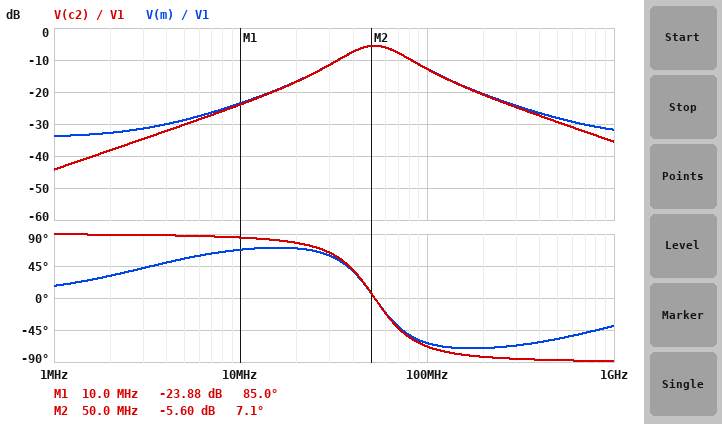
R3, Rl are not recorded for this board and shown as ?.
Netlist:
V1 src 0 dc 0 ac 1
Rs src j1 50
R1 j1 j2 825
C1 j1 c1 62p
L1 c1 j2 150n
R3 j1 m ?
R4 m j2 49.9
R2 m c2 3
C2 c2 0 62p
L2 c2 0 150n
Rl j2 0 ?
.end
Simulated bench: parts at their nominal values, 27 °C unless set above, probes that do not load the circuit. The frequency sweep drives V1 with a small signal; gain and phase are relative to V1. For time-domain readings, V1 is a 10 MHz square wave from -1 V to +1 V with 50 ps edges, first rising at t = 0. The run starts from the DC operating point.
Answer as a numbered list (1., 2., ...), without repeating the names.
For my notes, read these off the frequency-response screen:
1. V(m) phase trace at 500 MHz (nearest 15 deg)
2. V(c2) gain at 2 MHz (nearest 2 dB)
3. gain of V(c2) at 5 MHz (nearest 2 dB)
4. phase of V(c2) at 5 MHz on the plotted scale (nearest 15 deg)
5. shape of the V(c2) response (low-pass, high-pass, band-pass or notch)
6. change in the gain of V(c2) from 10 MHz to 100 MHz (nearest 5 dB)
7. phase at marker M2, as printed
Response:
1. -60 deg
2. -38 dB
3. -30 dB
4. 90 deg
5. band-pass
6. 10 dB
7. 7.1 deg
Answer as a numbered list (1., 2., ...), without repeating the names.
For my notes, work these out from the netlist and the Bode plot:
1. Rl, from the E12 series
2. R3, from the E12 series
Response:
1. 56 Ω
2. 100 Ω
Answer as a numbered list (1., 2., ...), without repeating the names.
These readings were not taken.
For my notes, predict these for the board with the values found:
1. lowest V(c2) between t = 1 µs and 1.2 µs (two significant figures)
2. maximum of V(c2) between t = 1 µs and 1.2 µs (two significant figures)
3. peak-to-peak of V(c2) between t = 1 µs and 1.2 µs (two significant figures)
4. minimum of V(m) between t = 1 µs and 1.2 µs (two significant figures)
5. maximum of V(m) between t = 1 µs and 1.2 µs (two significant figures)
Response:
1. -450 mV
2. 450 mV
3. 910 mV
4. -460 mV
5. 460 mV
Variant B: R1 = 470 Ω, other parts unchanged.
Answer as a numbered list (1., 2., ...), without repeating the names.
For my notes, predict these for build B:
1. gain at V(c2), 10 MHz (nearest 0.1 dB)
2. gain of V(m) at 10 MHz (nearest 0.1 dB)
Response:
1. -23.8 dB
2. -23.4 dB
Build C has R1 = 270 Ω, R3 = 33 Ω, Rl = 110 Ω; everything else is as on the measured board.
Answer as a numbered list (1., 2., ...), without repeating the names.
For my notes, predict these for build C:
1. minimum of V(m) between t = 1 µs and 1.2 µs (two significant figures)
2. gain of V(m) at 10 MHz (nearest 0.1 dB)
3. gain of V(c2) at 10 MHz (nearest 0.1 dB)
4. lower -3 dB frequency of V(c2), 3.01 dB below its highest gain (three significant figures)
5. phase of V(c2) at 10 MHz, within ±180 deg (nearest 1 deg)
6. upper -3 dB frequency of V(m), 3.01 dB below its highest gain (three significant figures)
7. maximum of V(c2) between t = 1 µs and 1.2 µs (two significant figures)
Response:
1. -680 mV
2. -18.7 dB
3. -19.1 dB
4. 34.8 MHz
5. 81 deg
6. 78.3 MHz
7. 680 mV
